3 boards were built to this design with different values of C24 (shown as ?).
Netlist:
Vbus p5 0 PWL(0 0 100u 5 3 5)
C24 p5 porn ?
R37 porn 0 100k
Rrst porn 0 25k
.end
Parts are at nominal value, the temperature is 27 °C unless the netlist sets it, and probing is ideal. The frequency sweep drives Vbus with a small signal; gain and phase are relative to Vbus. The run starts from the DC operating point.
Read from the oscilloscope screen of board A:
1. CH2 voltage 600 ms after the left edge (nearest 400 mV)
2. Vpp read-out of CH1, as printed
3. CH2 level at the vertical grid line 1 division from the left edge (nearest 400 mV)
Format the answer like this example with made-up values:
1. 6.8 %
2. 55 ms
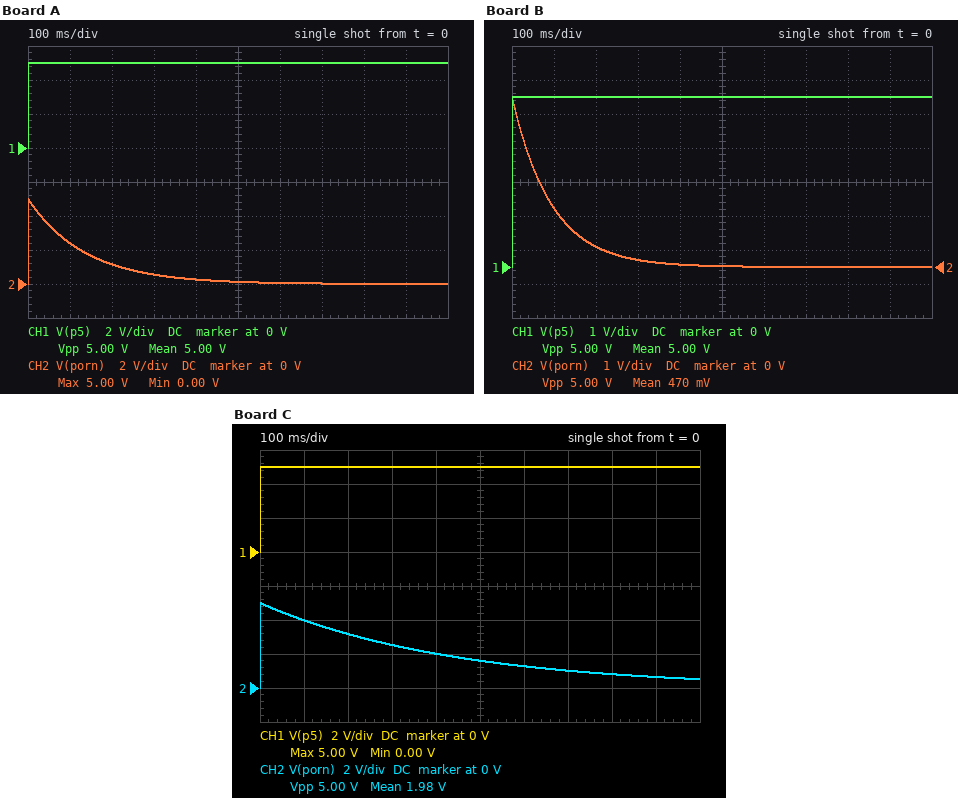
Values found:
1. 0 V
2. 5.00 V
3. 2.4 V
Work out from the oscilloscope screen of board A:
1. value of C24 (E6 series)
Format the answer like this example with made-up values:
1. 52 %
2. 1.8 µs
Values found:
1. 6.8 µF
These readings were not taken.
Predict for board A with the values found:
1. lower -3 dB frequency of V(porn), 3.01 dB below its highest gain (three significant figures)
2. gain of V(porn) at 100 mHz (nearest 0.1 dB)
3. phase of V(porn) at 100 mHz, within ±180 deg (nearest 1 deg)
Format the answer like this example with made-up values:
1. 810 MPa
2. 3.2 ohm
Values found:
1. 1.17 Hz
2. -21.4 dB
3. 85 deg
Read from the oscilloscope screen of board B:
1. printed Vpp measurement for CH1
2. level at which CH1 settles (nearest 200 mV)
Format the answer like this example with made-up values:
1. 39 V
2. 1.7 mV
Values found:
1. 5.00 V
2. 5.0 V
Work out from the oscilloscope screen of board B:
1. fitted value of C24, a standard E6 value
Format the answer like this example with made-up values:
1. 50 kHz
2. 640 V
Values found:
1. 4.7 µF
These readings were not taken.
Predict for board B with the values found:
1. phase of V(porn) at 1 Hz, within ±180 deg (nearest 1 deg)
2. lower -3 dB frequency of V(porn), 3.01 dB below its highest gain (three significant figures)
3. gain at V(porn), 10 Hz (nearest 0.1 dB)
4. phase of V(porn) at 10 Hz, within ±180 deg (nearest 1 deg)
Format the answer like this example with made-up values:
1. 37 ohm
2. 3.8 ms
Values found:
1. 59 deg
2. 1.69 Hz
3. -0.1 dB
4. 10 deg
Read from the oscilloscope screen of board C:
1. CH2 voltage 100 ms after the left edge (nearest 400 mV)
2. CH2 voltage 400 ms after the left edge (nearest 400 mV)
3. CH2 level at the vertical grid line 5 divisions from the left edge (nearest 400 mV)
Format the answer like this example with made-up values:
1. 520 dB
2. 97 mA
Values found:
1. 4.0 V
2. 2.0 V
3. 1.6 V
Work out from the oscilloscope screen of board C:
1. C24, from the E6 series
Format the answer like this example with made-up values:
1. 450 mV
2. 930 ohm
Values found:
1. 22 µF
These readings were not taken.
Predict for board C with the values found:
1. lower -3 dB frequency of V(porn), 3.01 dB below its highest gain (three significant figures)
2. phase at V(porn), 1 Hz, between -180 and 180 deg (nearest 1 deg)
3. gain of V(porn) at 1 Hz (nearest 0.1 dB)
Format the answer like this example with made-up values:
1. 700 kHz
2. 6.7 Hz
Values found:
1. 362 mHz
2. 20 deg
3. -0.5 dB
